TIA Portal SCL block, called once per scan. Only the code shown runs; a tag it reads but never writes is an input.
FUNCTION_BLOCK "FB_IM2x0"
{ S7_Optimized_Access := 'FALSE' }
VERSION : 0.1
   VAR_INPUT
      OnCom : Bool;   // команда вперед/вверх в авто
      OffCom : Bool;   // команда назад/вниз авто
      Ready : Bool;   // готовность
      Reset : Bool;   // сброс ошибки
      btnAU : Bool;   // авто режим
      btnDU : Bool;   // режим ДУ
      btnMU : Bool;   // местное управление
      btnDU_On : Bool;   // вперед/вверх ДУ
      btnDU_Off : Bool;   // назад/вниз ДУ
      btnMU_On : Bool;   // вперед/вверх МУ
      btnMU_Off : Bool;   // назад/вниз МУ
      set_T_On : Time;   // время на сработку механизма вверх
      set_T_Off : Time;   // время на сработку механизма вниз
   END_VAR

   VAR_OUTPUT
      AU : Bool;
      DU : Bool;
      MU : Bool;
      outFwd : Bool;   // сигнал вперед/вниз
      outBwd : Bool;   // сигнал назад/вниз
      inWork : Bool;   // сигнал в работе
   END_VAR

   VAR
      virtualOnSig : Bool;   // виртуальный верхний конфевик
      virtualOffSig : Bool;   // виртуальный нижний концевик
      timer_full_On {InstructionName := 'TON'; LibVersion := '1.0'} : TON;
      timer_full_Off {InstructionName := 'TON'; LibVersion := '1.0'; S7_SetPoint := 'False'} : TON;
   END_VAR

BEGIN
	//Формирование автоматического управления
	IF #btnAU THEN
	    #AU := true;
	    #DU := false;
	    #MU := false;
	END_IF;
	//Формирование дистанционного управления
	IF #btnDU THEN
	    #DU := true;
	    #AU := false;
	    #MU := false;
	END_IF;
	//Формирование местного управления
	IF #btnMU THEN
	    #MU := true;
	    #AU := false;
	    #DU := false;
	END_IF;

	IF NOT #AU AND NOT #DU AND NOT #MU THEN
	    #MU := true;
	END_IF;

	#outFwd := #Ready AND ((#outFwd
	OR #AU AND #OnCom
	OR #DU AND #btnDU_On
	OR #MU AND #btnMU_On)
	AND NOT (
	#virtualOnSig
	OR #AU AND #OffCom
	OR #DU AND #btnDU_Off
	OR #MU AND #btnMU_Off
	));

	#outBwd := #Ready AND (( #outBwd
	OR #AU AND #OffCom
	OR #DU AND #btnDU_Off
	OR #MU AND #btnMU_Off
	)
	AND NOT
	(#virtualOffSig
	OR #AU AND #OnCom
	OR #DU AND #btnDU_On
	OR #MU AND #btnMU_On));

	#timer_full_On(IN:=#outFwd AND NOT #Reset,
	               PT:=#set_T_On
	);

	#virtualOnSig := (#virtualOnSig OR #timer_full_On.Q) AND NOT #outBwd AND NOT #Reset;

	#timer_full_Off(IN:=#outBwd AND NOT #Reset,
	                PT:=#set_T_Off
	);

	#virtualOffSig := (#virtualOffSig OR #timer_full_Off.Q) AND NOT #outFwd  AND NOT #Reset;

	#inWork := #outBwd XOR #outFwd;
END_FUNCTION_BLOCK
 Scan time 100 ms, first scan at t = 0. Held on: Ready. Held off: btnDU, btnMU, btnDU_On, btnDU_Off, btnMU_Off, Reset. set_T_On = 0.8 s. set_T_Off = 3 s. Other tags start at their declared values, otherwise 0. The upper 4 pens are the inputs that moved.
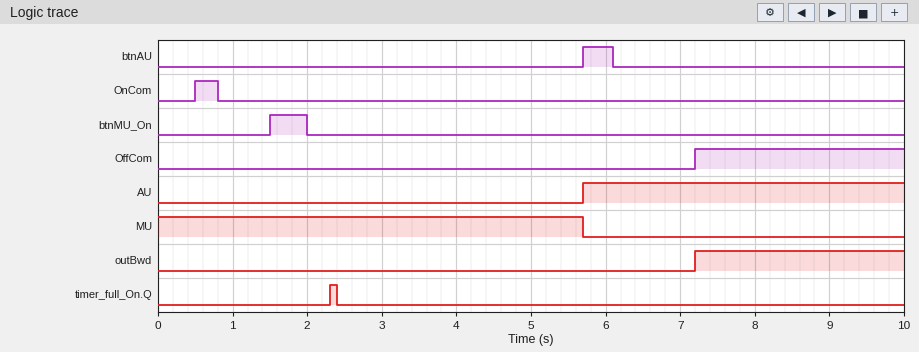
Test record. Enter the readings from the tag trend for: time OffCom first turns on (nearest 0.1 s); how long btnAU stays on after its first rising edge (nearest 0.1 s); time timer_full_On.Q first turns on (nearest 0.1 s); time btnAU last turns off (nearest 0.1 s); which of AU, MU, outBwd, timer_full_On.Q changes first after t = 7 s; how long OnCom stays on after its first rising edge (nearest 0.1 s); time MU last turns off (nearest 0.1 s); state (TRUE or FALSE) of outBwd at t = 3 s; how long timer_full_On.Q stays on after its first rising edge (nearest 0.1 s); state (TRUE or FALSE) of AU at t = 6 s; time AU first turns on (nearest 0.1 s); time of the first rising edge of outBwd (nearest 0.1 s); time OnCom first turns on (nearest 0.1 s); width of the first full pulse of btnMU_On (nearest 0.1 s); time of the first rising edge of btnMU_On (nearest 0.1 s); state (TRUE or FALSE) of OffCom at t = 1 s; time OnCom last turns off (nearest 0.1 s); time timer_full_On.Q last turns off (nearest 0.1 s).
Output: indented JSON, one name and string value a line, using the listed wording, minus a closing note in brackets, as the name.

{
  "time OffCom first turns on": "7.2 s",
  "how long btnAU stays on after its first rising edge": "0.4 s",
  "time timer_full_On.Q first turns on": "2.3 s",
  "time btnAU last turns off": "6.1 s",
  "which of AU, MU, outBwd, timer_full_On.Q changes first after t = 7 s": "outBwd",
  "how long OnCom stays on after its first rising edge": "0.3 s",
  "time MU last turns off": "5.7 s",
  "state (TRUE or FALSE) of outBwd at t = 3 s": "FALSE",
  "how long timer_full_On.Q stays on after its first rising edge": "0.1 s",
  "state (TRUE or FALSE) of AU at t = 6 s": "TRUE",
  "time AU first turns on": "5.7 s",
  "time of the first rising edge of outBwd": "7.2 s",
  "time OnCom first turns on": "0.5 s",
  "width of the first full pulse of btnMU_On": "0.5 s",
  "time of the first rising edge of btnMU_On": "1.5 s",
  "state (TRUE or FALSE) of OffCom at t = 1 s": "FALSE",
  "time OnCom last turns off": "0.8 s",
  "time timer_full_On.Q last turns off": "2.4 s"
}
